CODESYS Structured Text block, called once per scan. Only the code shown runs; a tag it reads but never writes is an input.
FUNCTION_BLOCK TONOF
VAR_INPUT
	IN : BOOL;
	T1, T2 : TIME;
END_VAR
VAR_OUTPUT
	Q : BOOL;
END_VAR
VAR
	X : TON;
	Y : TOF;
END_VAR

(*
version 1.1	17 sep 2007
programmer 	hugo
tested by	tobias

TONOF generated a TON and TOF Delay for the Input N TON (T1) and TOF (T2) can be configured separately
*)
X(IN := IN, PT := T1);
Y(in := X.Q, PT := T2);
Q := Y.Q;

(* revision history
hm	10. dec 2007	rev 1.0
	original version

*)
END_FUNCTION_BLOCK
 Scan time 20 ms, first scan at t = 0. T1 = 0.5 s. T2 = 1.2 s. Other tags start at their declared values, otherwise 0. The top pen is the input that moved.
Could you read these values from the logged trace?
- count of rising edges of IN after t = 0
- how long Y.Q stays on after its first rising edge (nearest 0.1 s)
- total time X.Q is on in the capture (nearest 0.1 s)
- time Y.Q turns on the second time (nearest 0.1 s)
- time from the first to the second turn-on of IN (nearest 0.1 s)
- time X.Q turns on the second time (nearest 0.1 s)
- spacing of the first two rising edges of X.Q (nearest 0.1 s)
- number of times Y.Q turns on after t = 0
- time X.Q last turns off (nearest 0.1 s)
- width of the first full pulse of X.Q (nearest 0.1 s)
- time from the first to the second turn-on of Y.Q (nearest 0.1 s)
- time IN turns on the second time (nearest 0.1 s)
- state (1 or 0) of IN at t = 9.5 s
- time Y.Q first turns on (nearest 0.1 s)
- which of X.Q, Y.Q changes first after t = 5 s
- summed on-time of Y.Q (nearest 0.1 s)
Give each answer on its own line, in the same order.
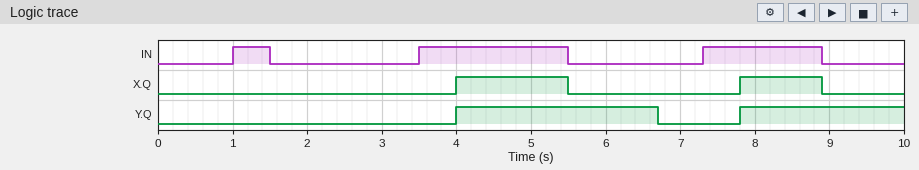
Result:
3
2.7 s
2.6 s
7.8 s
2.5 s
7.8 s
3.8 s
2
8.9 s
1.5 s
3.8 s
3.5 s
0
4.0 s
X.Q
4.9 s
